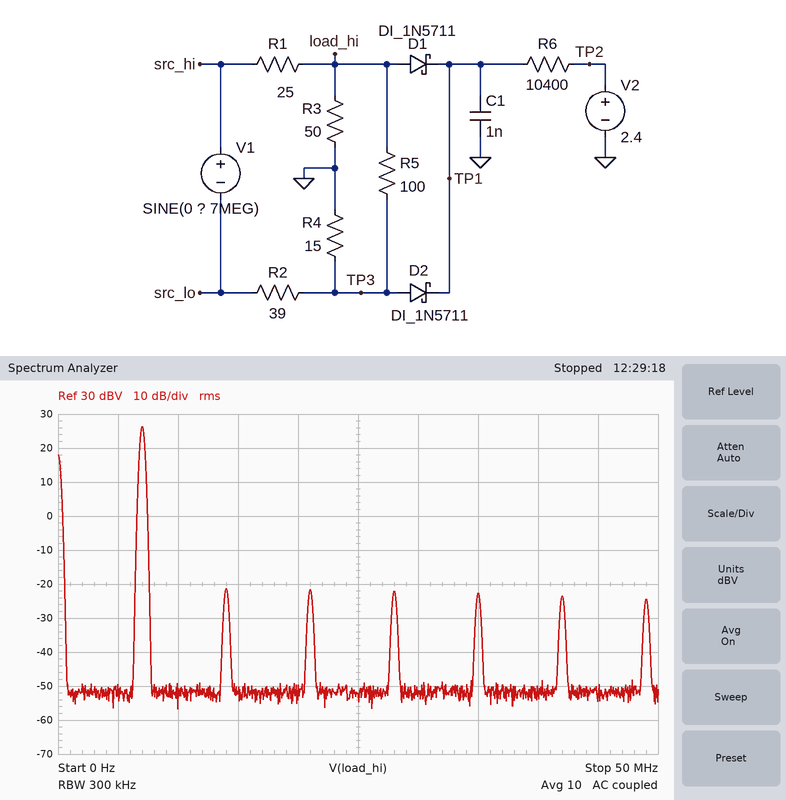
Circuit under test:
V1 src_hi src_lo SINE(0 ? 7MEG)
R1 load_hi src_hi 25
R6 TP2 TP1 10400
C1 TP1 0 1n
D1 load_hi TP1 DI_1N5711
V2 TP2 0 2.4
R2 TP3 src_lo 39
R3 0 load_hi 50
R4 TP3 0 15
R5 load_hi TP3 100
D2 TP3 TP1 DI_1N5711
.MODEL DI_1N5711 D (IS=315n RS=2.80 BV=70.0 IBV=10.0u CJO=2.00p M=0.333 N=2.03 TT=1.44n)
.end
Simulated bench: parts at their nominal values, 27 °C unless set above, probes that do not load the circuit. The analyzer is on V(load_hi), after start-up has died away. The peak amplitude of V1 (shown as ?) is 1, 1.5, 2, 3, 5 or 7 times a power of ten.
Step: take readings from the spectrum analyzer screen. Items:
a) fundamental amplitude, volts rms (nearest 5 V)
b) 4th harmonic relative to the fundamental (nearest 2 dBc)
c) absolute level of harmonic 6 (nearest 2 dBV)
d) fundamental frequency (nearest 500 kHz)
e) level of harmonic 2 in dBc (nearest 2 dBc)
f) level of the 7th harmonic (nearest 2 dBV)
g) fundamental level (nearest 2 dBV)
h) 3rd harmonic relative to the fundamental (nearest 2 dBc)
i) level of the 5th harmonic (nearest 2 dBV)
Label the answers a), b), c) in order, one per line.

a) 20 V
b) -48 dBc
c) -24 dBV
d) 7.0 MHz
e) -48 dBc
f) -24 dBV
g) 26 dBV
h) -48 dBc
i) -22 dBV
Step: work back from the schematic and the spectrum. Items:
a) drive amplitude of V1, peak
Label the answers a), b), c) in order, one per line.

a) 100 V
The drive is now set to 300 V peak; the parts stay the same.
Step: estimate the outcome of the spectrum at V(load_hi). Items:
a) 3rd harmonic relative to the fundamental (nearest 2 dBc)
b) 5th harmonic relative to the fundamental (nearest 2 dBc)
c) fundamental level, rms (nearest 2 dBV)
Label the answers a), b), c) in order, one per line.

a) -16 dBc
b) -24 dBc
c) 32 dBV
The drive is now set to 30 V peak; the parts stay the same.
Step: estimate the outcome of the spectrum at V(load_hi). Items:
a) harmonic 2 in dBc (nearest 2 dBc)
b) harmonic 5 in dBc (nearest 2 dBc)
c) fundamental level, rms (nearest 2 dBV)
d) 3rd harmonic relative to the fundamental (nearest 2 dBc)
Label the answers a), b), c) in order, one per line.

a) -50 dBc
b) -52 dBc
c) 16 dBV
d) -50 dBc
